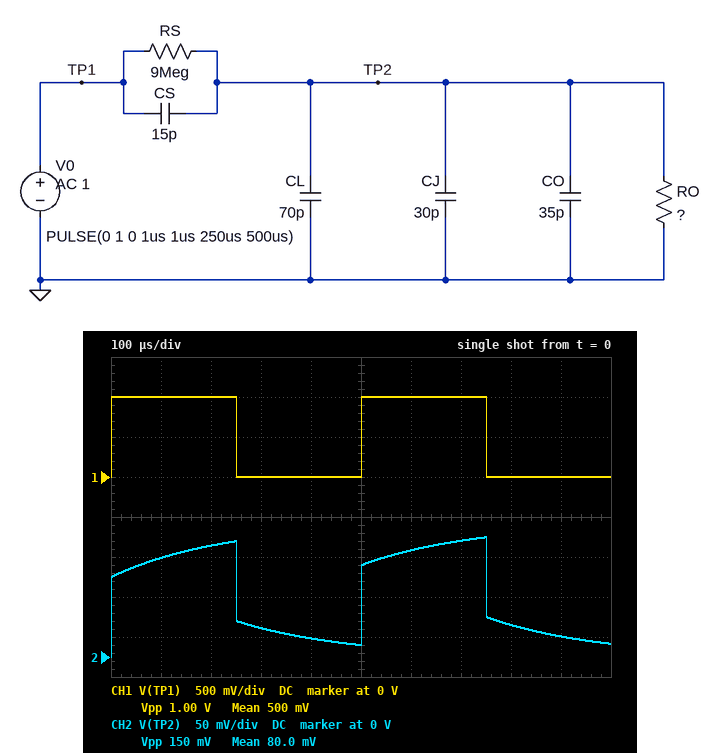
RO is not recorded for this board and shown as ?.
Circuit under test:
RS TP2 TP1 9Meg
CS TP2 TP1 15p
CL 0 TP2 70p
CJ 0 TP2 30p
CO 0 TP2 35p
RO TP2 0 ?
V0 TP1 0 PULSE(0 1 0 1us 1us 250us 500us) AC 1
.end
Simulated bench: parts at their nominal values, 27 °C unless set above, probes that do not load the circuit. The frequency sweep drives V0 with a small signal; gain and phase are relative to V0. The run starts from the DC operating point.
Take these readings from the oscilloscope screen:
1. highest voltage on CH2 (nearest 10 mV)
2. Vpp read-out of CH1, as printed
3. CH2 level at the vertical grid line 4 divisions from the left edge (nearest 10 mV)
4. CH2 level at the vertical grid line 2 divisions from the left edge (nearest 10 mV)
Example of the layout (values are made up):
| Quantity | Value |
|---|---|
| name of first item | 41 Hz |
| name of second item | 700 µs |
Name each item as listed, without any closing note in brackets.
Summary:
| Quantity | Value |
|---|---|
| highest voltage on CH2 | 150 mV |
| Vpp read-out of CH1, as printed | 1.00 V |
| CH2 level at the vertical grid line 4 divisions from the left edge | 20 mV |
| CH2 level at the vertical grid line 2 divisions from the left edge | 140 mV |
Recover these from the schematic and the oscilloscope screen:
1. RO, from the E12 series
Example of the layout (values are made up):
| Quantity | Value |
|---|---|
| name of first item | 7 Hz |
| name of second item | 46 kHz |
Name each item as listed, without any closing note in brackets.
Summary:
| Quantity | Value |
|---|---|
| RO, from the E12 series | 1.8 MΩ |
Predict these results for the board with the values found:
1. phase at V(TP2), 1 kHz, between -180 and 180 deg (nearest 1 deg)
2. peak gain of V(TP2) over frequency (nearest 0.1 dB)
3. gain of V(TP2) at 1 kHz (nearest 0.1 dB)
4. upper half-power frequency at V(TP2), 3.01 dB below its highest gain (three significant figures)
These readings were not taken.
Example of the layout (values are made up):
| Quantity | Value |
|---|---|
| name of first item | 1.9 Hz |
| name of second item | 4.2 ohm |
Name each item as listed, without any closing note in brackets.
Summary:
| Quantity | Value |
|---|---|
| phase at V(TP2), 1 kHz, between -180 and 180 deg | -14 deg |
| peak gain of V(TP2) over frequency | -15.6 dB |
| gain of V(TP2) at 1 kHz | -18.0 dB |
| upper half-power frequency at V(TP2), 3.01 dB below its highest gain | 1.34 kHz |
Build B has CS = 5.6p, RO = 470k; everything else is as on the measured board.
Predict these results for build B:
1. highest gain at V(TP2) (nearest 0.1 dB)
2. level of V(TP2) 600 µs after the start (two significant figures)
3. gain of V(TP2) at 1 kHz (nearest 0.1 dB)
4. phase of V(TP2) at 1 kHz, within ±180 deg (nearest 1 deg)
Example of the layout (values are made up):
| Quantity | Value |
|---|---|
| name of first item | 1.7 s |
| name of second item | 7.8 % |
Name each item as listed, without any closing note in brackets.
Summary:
| Quantity | Value |
|---|---|
| highest gain at V(TP2) | -26.1 dB |
| level of V(TP2) 600 µs after the start | 48 mV |
| gain of V(TP2) at 1 kHz | -26.3 dB |
| phase of V(TP2) at 1 kHz, within ±180 deg | -4 deg |
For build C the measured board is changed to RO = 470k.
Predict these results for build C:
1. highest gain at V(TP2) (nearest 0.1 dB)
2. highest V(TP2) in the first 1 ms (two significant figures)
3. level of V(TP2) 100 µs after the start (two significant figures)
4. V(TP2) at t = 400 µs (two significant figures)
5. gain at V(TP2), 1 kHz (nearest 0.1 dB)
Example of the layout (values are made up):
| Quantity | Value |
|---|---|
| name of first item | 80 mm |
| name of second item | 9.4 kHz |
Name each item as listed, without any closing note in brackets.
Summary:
| Quantity | Value |
|---|---|
| highest gain at V(TP2) | -20.0 dB |
| highest V(TP2) in the first 1 ms | 100 mV |
| level of V(TP2) 100 µs after the start | 61 mV |
| V(TP2) at t = 400 µs | -5.4 mV |
| gain at V(TP2), 1 kHz | -24.4 dB |
